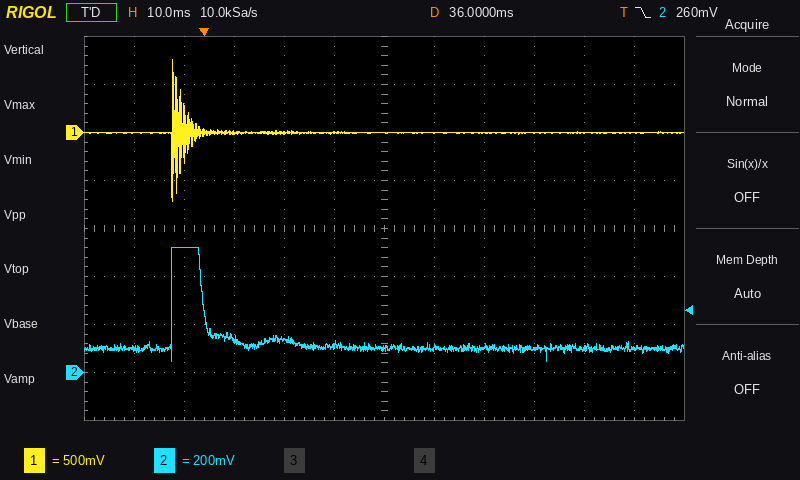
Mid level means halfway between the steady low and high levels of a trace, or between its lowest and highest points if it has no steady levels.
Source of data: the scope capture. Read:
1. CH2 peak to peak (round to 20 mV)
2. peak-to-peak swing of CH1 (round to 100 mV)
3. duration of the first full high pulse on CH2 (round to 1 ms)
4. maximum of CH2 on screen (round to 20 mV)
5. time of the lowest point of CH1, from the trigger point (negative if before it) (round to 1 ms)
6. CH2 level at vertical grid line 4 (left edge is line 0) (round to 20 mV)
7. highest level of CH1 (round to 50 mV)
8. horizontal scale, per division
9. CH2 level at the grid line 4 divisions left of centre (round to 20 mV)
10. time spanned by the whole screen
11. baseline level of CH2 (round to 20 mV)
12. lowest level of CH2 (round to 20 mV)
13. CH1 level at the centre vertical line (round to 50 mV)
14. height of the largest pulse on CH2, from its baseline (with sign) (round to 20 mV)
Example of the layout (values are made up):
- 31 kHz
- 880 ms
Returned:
- 480 mV
- 1.50 V
- 6 ms
- 520 mV
- -6 ms
- 140 mV
- 750 mV
- 10 ms
- 520 mV
- 120 ms
- 100 mV
- 40 mV
- 0 mV
- +420 mV
